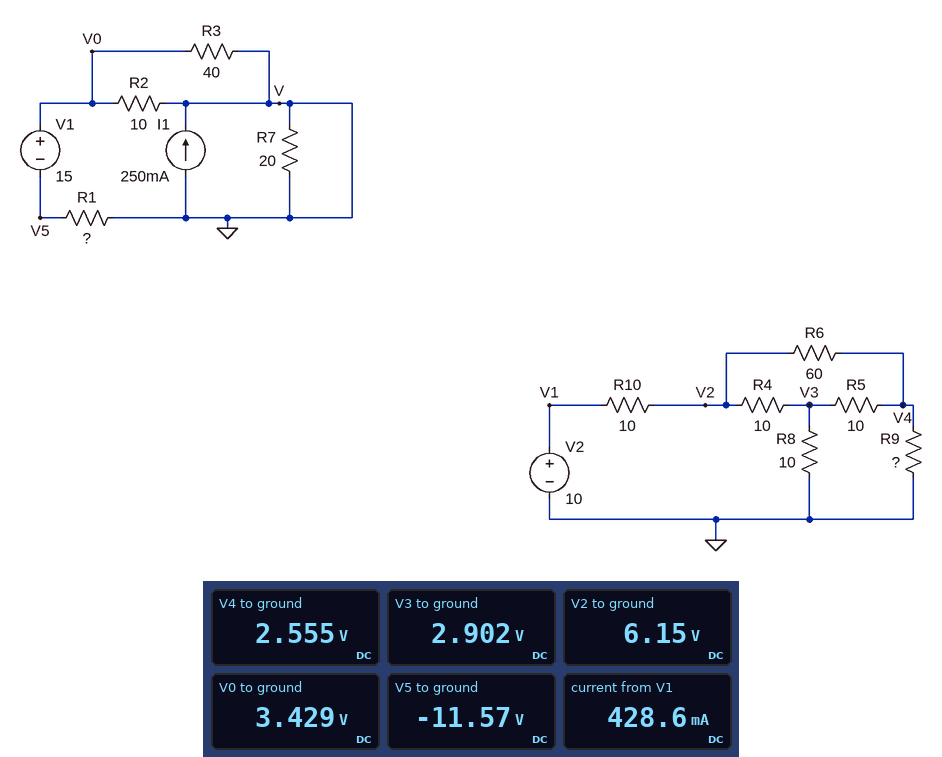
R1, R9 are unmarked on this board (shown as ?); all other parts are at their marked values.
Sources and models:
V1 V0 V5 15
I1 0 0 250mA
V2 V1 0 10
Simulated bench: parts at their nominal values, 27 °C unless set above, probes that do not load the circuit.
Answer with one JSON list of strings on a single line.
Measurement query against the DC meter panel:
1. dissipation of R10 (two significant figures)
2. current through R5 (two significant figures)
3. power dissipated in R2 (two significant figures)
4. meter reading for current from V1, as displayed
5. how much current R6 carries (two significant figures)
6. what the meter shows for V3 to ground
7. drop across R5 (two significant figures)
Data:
["1.5 W", "35 mA", "1.2 W", "428.6 mA", "60 mA", "2.902 V", "350 mV"]
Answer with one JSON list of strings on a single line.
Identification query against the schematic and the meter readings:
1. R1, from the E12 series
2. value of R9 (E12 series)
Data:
["27 Ω", "27 Ω"]
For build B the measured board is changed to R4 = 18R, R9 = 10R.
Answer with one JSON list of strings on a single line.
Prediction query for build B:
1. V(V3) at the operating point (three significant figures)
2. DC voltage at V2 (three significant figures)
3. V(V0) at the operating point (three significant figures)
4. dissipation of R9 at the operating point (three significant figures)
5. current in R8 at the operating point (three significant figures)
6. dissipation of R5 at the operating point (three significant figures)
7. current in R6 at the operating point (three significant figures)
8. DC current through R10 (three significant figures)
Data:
["1.99 V", "6.59 V", "3.43 V", "203 mW", "199 mA", "31.9 mW", "86.0 mA", "341 mA"]
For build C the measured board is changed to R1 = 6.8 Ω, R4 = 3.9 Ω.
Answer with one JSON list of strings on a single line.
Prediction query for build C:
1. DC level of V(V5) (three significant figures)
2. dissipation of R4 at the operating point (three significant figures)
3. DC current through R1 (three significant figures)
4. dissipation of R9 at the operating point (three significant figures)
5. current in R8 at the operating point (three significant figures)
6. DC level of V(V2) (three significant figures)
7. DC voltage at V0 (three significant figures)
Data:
["-6.89 V", "724 mW", "1.01 A", "318 mW", "362 mA", "5.30 V", "8.11 V"]
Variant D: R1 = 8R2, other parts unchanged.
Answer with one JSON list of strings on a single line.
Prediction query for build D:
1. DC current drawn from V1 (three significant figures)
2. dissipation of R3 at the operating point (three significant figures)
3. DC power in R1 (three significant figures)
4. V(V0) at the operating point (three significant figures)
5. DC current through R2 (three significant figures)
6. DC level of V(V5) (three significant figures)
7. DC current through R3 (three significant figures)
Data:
["926 mA", "1.37 W", "7.03 W", "7.41 V", "741 mA", "-7.59 V", "185 mA"]
